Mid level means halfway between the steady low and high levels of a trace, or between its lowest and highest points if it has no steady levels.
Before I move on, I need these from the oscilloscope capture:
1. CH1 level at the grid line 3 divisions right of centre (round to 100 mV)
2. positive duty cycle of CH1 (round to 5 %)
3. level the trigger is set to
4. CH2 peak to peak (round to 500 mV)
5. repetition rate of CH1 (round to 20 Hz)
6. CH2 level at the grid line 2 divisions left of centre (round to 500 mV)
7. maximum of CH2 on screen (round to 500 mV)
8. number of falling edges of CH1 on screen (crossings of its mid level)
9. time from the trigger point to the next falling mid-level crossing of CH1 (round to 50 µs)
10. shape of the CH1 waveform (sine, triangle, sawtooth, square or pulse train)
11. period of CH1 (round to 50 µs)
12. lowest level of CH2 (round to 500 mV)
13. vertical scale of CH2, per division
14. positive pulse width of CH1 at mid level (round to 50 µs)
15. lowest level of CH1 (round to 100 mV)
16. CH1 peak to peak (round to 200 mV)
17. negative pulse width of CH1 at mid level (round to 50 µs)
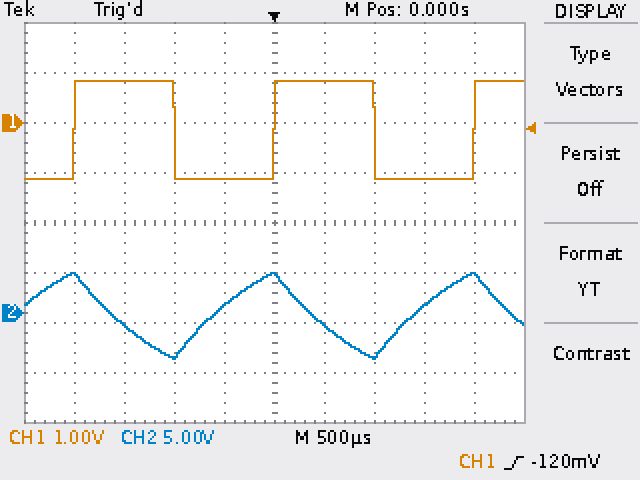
-1.1 V
50 %
-120 mV
8.5 V
500 Hz
-4.5 V
4.0 V
2
1.00 ms
square
2.00 ms
-4.5 V
5 V
1.00 ms
-1.1 V
2.0 V
1.00 ms
